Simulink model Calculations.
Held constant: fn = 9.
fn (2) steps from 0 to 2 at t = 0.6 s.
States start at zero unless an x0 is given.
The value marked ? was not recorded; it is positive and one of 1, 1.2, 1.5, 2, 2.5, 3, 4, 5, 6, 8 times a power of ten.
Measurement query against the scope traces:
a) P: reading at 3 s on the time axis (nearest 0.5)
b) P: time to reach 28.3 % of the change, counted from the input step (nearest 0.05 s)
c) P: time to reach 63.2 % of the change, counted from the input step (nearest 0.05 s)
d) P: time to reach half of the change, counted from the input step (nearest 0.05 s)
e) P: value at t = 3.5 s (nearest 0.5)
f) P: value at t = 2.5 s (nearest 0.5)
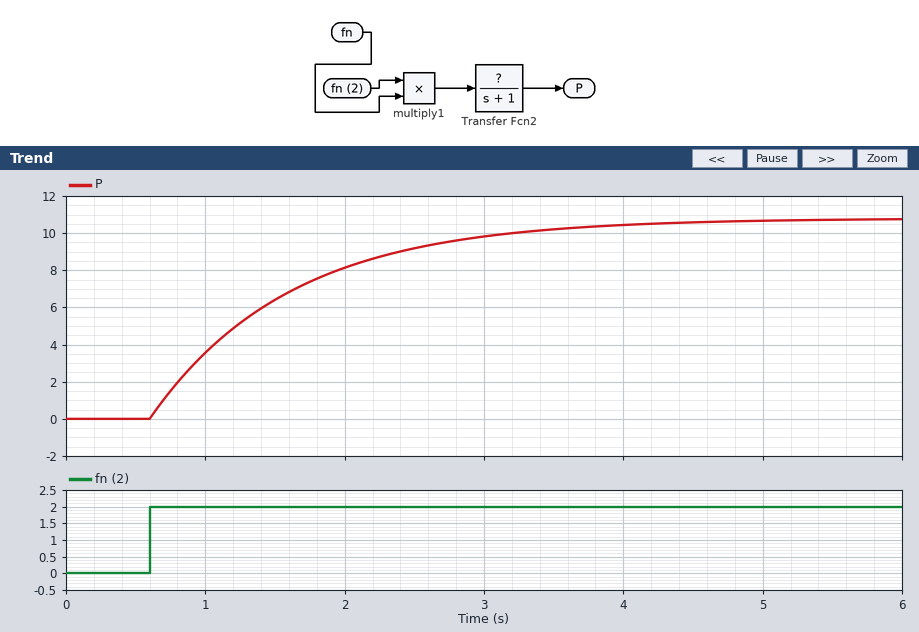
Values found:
10.0
0.35 s
1.00 s
0.70 s
10.0
9.0
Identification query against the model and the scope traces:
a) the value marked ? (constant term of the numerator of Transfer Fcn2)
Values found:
0.6
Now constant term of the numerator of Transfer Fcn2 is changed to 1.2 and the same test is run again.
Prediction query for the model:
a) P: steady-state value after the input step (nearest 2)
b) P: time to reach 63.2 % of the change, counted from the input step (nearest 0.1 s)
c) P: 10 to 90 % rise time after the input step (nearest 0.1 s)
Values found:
22
1.0 s
2.2 s
